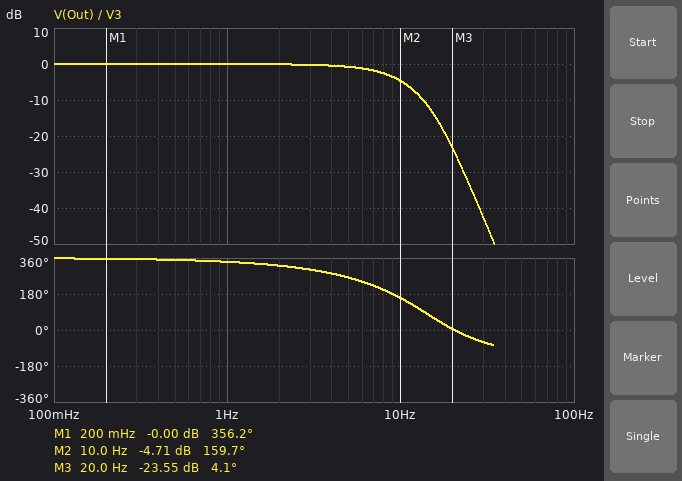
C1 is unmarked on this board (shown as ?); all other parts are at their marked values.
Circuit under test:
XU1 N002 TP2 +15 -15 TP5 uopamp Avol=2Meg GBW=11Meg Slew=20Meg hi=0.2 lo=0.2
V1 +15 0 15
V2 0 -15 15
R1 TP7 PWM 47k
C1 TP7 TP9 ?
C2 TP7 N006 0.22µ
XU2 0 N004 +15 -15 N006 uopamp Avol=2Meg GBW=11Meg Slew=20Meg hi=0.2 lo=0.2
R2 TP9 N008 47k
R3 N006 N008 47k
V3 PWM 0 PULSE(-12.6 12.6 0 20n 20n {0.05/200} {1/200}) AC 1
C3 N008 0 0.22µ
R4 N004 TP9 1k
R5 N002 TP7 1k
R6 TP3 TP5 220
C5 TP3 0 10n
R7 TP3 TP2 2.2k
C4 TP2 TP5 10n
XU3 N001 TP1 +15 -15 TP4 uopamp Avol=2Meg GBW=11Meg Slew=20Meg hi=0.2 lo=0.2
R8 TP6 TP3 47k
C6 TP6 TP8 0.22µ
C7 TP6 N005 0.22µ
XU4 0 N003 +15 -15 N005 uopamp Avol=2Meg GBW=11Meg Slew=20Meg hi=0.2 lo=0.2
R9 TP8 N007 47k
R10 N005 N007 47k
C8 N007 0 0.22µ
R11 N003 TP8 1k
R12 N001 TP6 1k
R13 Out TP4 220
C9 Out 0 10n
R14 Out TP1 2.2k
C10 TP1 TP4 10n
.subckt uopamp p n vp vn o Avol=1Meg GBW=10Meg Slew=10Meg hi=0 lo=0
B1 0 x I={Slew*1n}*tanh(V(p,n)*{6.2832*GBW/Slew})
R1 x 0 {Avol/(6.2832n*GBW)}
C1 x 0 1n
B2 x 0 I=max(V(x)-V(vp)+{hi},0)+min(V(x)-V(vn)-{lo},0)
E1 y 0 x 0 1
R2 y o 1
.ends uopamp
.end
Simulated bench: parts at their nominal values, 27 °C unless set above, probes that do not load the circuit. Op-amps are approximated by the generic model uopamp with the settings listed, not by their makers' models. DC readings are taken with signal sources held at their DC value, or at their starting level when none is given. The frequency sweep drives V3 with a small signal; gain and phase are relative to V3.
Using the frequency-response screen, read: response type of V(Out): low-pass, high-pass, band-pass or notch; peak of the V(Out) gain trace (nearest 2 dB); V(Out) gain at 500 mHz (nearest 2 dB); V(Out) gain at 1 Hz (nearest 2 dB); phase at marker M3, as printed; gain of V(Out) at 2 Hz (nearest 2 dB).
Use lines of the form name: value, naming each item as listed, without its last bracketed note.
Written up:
response type of V(Out): low-pass, high-pass, band-pass or notch: low-pass
peak of the V(Out) gain trace: 0 dB
V(Out) gain at 500 mHz: 0 dB
V(Out) gain at 1 Hz: 0 dB
phase at marker M3, as printed: 4.1 deg
gain of V(Out) at 2 Hz: 0 dB
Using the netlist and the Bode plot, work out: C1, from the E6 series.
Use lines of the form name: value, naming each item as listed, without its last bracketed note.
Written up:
C1, from the E6 series: 470 nF
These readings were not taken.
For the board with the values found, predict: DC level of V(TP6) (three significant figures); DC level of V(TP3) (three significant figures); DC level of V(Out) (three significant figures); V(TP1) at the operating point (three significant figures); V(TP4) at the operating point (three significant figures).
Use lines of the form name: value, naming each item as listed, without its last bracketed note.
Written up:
DC level of V(TP6): -12.6 V
DC level of V(TP3): -12.6 V
DC level of V(Out): -12.6 V
V(TP1) at the operating point: -12.6 V
V(TP4) at the operating point: -12.6 V
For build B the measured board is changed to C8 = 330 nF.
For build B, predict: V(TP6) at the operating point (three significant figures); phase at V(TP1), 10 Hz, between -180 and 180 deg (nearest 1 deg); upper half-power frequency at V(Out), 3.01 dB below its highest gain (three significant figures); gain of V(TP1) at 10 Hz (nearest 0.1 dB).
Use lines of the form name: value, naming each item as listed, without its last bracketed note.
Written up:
V(TP6) at the operating point: -12.6 V
phase at V(TP1), 10 Hz, between -180 and 180 deg: 161 deg
upper half-power frequency at V(Out), 3.01 dB below its highest gain: 9.38 Hz
gain of V(TP1) at 10 Hz: -3.5 dB
